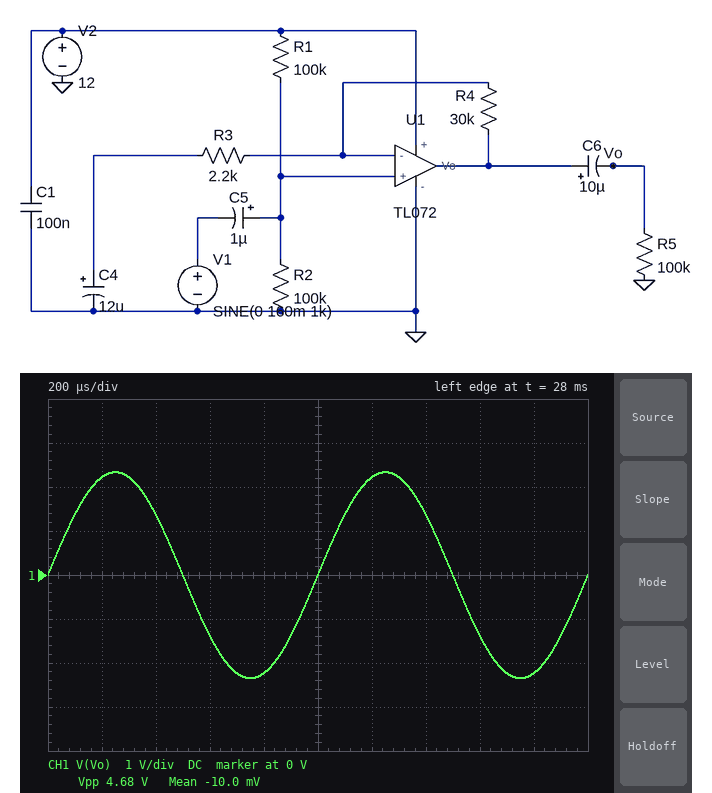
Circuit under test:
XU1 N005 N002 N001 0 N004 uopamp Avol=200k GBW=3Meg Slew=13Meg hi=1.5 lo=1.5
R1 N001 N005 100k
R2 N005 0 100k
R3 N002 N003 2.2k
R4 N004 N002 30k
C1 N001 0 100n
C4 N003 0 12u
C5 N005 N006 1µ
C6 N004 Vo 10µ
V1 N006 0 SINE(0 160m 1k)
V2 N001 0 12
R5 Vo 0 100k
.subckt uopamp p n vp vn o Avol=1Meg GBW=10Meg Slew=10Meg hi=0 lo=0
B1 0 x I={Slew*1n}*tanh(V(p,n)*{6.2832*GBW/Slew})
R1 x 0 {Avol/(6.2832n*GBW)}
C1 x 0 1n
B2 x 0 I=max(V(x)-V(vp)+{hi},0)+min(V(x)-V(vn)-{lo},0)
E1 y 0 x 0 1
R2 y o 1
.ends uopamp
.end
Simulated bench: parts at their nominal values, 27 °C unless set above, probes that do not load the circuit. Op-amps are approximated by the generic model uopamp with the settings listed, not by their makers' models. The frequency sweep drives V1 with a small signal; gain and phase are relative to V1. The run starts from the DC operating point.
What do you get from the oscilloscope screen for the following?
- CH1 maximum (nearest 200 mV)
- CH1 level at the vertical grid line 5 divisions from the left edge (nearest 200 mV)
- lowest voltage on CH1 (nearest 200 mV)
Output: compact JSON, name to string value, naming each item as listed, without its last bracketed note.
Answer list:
{"CH1 maximum": "2.4 V", "CH1 level at the vertical grid line 5 divisions from the left edge": "0 V", "lowest voltage on CH1": "-2.4 V"}
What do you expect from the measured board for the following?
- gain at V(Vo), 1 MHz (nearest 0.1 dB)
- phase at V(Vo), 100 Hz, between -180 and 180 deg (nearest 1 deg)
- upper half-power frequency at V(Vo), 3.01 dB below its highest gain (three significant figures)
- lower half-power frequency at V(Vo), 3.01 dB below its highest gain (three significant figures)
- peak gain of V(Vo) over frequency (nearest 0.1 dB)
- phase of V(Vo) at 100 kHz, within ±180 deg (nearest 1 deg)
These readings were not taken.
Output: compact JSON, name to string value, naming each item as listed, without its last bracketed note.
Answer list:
{"gain at V(Vo), 1 MHz": "9.4 dB", "phase at V(Vo), 100 Hz, between -180 and 180 deg": "5 deg", "upper half-power frequency at V(Vo), 3.01 dB below its highest gain": "205 kHz", "lower half-power frequency at V(Vo), 3.01 dB below its highest gain": "7.29 Hz", "peak gain of V(Vo) over frequency": "23.3 dB", "phase of V(Vo) at 100 kHz, within ±180 deg": "-26 deg"}
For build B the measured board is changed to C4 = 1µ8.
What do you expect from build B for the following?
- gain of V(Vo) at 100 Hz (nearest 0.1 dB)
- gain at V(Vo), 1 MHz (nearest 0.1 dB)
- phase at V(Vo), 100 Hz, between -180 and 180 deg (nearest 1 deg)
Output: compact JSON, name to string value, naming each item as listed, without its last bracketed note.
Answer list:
{"gain of V(Vo) at 100 Hz": "22.7 dB", "gain at V(Vo), 1 MHz": "9.4 dB", "phase at V(Vo), 100 Hz, between -180 and 180 deg": "22 deg"}
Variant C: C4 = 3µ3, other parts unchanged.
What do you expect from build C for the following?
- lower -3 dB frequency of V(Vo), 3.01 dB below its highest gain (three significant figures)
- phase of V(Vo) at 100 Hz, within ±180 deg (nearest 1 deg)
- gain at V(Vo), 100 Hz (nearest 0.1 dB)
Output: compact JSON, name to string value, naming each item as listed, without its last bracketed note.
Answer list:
{"lower -3 dB frequency of V(Vo), 3.01 dB below its highest gain": "22.3 Hz", "phase of V(Vo) at 100 Hz, within ±180 deg": "13 deg", "gain at V(Vo), 100 Hz": "23.1 dB"}
